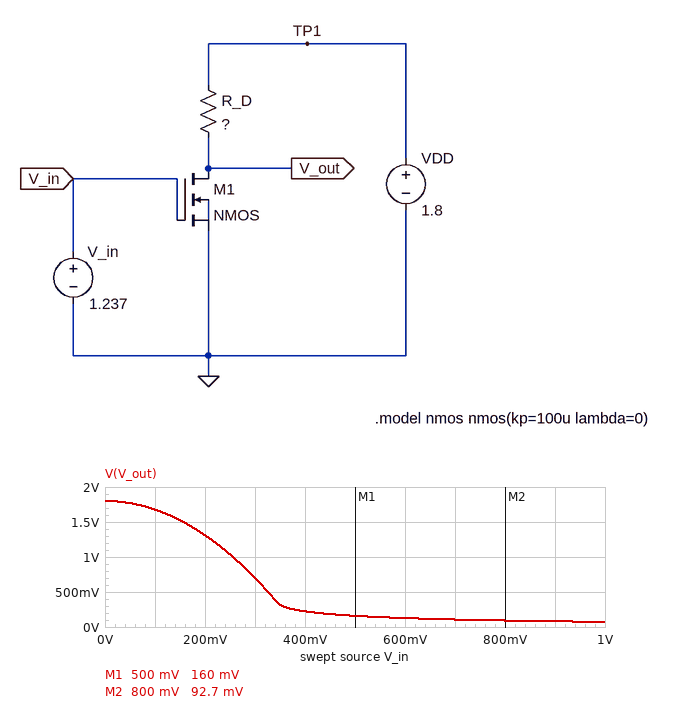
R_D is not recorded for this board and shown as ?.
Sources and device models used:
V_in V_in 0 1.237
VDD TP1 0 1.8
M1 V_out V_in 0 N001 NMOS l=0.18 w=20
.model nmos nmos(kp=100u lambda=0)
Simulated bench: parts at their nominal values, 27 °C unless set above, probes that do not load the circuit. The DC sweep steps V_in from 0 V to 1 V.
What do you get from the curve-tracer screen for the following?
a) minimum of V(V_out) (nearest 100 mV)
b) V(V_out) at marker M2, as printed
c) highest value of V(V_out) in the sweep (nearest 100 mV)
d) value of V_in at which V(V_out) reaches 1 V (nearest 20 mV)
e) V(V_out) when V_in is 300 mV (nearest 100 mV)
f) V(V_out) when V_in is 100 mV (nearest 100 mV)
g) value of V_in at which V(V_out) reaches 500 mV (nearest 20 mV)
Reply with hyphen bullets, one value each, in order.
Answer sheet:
- 100 mV
- 92.7 mV
- 1.8 V
- 260 mV
- 700 mV
- 1.7 V
- 320 mV
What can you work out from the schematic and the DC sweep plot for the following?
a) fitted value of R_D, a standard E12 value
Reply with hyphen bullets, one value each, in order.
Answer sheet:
- 2.2 kΩ
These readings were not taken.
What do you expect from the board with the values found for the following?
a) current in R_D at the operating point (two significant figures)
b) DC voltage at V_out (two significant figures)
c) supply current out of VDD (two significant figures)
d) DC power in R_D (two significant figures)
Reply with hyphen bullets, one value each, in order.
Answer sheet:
- 790 µA
- 59 mV
- 790 µA
- 1.4 mW
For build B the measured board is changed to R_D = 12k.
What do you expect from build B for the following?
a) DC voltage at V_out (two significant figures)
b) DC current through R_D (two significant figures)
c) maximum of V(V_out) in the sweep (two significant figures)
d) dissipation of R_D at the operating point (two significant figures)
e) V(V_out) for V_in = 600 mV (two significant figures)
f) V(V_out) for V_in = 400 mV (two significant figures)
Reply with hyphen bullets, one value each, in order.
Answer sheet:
- 11 mV
- 150 µA
- 1.8 V
- 270 µW
- 23 mV
- 35 mV
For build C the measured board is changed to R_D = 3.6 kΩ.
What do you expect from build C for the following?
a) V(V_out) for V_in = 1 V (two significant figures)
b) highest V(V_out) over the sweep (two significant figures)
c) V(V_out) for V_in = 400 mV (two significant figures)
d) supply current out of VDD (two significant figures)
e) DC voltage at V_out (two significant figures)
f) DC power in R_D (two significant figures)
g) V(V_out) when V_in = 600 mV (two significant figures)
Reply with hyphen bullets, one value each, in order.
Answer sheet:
- 45 mV
- 1.8 V
- 120 mV
- 490 µA
- 36 mV
- 860 µW
- 77 mV
